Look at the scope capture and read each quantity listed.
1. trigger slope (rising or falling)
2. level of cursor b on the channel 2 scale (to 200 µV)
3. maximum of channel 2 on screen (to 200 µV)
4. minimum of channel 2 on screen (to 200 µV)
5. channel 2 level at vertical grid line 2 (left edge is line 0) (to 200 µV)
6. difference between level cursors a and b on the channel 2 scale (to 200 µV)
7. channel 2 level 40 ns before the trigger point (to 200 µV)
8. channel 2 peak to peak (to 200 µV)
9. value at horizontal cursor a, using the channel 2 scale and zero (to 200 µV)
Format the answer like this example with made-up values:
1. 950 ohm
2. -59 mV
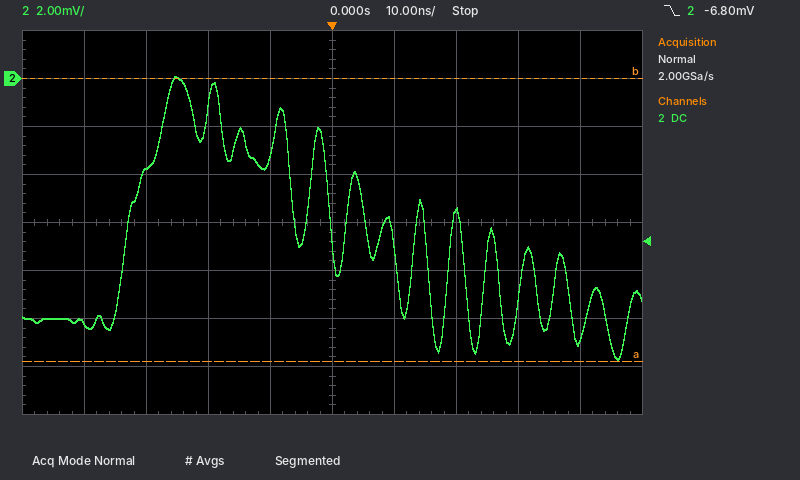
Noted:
1. falling
2. 0.0 mV
3. 0.0 mV
4. -11.8 mV
5. -3.8 mV
6. 11.8 mV
7. -10.2 mV
8. 11.8 mV
9. -11.8 mV
